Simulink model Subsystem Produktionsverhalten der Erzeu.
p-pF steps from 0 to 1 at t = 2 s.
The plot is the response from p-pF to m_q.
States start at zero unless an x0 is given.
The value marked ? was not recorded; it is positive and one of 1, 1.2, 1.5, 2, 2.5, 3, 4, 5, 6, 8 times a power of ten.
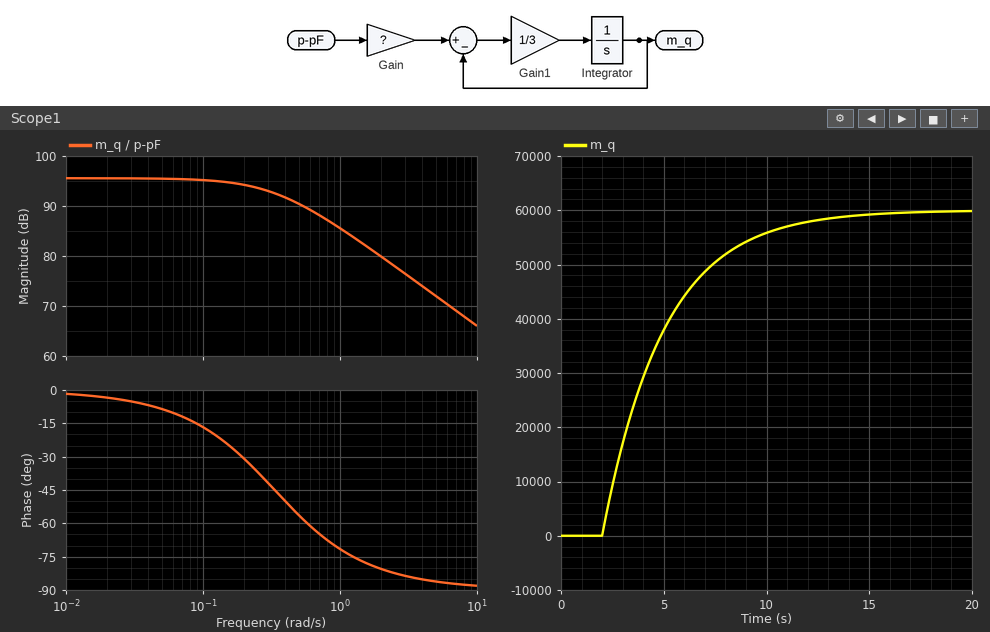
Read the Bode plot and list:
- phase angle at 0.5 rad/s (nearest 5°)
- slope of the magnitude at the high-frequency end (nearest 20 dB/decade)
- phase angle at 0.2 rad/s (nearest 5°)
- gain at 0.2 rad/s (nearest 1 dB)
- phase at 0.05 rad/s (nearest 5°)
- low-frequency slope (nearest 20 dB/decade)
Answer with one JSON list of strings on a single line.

["-55°", "-20 dB/decade", "-30°", "94 dB", "-10°", "0 dB/decade"]
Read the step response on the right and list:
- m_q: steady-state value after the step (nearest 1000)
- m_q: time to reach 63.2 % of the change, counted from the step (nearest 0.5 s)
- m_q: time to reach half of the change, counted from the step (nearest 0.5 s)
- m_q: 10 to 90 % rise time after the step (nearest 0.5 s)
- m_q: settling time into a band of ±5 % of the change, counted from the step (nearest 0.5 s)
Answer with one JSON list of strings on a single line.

["60000", "3.0 s", "2.0 s", "6.5 s", "9.0 s"]
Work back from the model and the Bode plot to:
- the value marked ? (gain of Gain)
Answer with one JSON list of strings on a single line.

["60000"]
